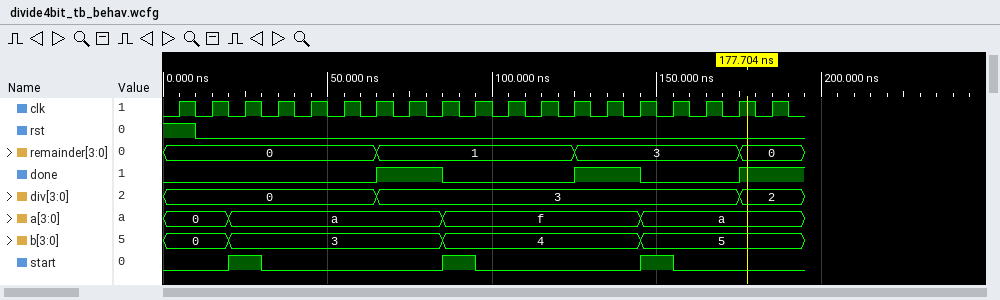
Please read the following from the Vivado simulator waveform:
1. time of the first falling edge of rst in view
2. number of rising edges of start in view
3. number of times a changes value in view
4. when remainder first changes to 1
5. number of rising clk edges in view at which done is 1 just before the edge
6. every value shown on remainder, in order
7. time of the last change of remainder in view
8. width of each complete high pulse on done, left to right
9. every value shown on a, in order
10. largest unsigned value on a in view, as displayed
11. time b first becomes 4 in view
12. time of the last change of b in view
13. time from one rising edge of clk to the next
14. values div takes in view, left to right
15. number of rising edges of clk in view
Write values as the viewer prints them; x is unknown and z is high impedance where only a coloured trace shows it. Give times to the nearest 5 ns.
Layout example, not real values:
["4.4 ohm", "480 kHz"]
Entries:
["10 ns", "3", "3", "65 ns", "5", "0, 1, 3, 0", "175 ns", "20 ns, 20 ns", "0, a, f, a", "f", "85 ns", "145 ns", "10 ns", "0, 3, 2", "19"]
